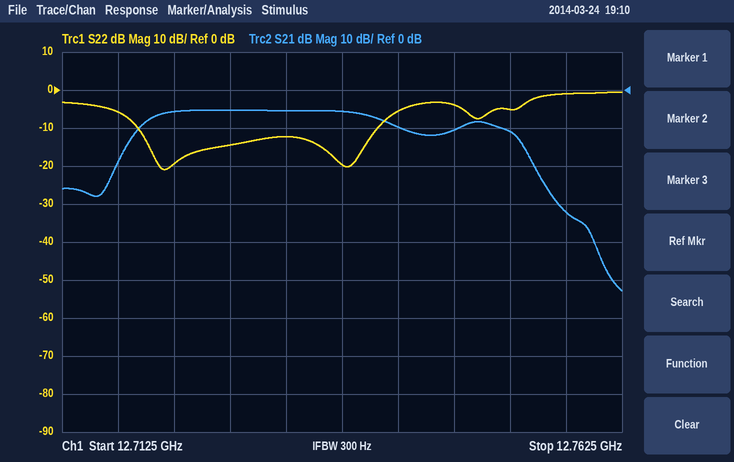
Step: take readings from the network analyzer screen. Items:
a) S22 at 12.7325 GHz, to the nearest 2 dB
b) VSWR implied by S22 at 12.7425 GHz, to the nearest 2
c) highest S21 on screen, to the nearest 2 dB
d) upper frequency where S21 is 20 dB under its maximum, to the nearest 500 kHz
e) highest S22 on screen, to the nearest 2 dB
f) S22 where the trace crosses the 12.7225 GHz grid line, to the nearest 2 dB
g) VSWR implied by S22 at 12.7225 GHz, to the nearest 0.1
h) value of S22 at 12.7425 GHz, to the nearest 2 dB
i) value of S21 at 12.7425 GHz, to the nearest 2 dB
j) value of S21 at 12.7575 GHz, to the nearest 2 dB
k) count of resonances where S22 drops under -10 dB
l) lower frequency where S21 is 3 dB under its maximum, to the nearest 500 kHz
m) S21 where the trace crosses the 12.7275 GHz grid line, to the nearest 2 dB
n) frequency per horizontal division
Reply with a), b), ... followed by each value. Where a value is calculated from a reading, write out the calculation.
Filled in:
a) -12 dB
b) |Γ| = 10^(-6/20) = 0.5012; VSWR = (1 + 0.5012)/(1 − 0.5012) ≈ 3.01, so 4 to the nearest 2
c) -6 dB
d) 12.7555 GHz
e) 0 dB
f) -20 dB
g) |Γ| = 10^(-20/20) = 0.1000; VSWR = (1 + 0.1000)/(1 − 0.1000) ≈ 1.2
h) -6 dB
i) -10 dB
j) -32 dB
k) 2
l) 12.7200 GHz
m) -6 dB
n) 5 MHz
